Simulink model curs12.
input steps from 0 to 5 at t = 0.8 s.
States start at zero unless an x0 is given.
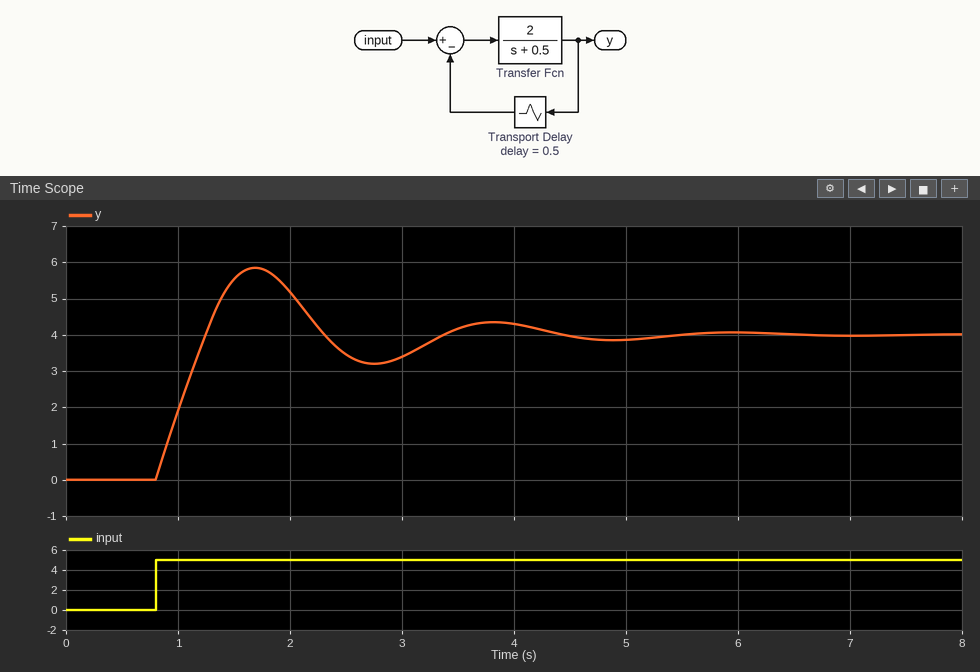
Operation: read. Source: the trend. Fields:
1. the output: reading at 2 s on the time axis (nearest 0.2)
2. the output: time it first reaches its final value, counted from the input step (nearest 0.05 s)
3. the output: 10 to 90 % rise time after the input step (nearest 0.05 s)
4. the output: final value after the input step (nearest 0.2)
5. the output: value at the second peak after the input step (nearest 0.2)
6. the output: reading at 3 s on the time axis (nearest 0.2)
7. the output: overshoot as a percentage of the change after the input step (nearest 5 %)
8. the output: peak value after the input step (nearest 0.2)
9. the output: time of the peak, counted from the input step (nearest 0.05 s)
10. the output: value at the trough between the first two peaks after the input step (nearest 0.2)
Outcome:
5.2
0.45 s
0.35 s
4.0
4.4
3.4
45 %
5.8
0.90 s
3.2
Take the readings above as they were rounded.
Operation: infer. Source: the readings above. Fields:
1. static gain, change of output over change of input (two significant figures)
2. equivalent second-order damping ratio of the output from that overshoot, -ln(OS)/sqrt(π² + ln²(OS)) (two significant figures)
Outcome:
0.80
0.25
